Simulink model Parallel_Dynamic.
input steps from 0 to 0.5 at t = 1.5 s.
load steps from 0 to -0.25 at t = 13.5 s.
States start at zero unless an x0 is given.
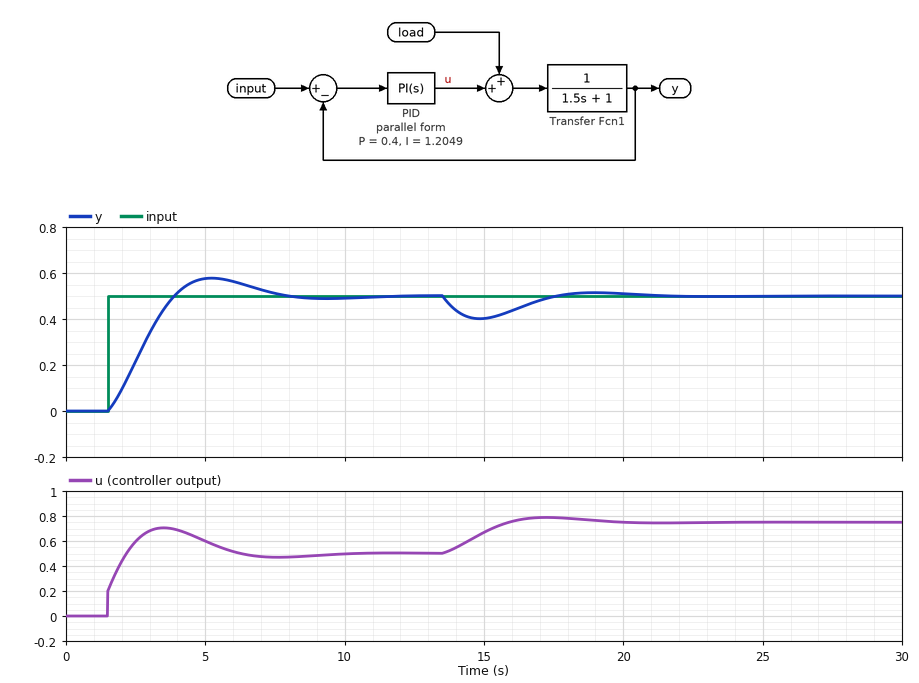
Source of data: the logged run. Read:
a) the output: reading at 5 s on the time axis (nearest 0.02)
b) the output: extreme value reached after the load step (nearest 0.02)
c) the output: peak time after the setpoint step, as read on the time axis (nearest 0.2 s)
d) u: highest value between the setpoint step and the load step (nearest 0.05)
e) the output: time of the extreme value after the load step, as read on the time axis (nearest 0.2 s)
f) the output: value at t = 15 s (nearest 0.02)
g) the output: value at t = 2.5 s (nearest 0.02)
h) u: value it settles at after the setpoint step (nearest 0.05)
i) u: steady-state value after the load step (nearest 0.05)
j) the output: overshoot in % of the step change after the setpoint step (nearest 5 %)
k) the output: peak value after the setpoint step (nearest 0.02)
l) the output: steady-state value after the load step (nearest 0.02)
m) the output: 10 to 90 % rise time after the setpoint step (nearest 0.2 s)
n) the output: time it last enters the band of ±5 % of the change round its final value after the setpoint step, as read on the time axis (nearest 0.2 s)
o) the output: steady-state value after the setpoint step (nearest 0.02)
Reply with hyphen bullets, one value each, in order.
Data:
- 0.58
- 0.40
- 5.2 s
- 0.70
- 14.8 s
- 0.40
- 0.22
- 0.50
- 0.75
- 15 %
- 0.58
- 0.50
- 1.8 s
- 7.0 s
- 0.50
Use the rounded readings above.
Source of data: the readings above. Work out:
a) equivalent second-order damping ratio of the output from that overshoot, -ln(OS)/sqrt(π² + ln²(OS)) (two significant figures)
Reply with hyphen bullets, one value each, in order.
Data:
- 0.52
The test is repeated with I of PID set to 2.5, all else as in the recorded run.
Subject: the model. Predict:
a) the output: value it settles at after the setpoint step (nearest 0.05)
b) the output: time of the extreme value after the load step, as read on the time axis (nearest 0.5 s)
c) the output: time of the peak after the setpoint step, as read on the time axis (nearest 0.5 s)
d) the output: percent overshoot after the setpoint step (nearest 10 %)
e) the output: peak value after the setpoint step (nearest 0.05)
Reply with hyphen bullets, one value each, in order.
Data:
- 0.50
- 14.5 s
- 4.0 s
- 30 %
- 0.65
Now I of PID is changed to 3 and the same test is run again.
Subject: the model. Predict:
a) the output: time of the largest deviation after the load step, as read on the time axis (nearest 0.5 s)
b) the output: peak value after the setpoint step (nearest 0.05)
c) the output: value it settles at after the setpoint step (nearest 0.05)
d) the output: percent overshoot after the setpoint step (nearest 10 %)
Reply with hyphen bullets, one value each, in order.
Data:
- 14.5 s
- 0.65
- 0.50
- 30 %
